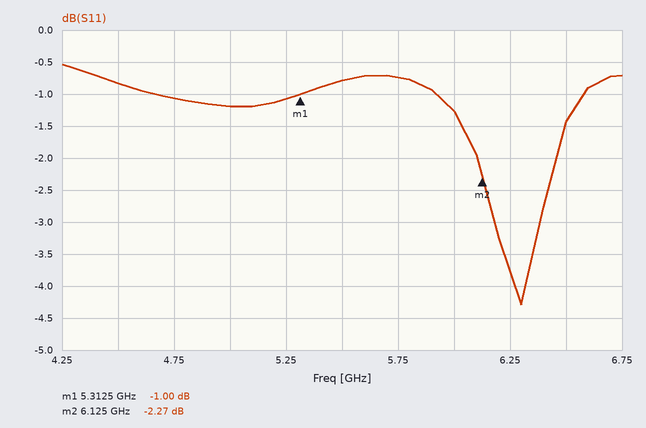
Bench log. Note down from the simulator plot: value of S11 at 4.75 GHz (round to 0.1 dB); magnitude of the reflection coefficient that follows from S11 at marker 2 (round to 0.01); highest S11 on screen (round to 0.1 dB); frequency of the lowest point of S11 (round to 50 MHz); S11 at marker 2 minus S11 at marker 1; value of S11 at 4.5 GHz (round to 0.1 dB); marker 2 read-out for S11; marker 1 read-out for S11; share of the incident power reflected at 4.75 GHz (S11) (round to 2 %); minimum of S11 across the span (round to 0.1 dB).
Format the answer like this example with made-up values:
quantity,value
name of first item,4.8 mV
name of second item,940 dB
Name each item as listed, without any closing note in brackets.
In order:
quantity,value
value of S11 at 4.75 GHz,-1.1 dB
magnitude of the reflection coefficient that follows from S11 at marker 2,0.77
highest S11 on screen,-0.5 dB
frequency of the lowest point of S11,6.30 GHz
S11 at marker 2 minus S11 at marker 1,-1.27 dB
value of S11 at 4.5 GHz,-0.8 dB
marker 2 read-out for S11,-2.27 dB
marker 1 read-out for S11,-1.00 dB
share of the incident power reflected at 4.75 GHz (S11),78 %
minimum of S11 across the span,-4.3 dB
